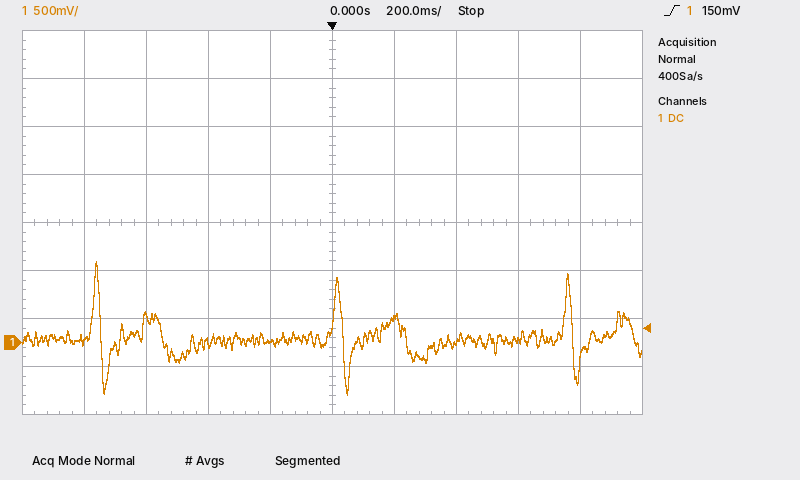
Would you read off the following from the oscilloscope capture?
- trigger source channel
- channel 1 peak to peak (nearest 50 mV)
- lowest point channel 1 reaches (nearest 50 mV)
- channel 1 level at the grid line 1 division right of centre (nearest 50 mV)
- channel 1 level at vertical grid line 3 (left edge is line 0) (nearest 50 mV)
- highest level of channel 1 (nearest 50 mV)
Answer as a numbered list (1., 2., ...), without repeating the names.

1. channel 1
2. 1.40 V
3. -550 mV
4. 250 mV
5. 0 mV
6. 850 mV
